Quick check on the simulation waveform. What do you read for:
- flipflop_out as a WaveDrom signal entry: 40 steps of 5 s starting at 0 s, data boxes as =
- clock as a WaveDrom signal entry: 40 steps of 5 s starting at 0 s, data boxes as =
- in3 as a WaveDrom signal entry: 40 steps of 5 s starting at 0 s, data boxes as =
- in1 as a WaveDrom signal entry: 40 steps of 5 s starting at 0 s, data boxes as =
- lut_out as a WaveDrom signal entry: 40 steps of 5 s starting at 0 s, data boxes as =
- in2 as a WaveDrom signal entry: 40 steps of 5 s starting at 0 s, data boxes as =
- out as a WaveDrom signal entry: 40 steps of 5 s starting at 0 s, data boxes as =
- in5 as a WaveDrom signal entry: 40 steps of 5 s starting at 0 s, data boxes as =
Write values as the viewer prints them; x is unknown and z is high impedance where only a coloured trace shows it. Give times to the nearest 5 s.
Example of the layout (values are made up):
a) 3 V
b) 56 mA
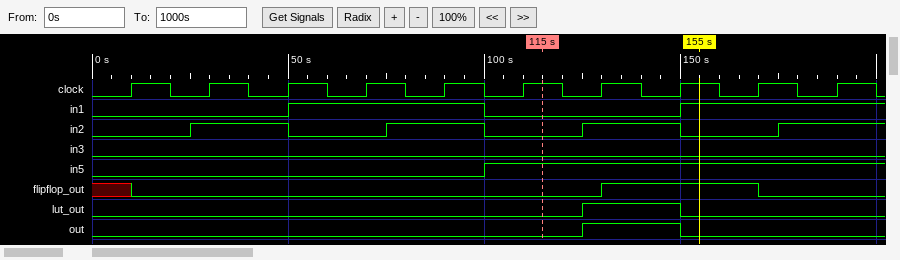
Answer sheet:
a) {name: 'flipflop_out', wave: 'x.0.......................1.......0.....'}
b) {name: 'clock', wave: '0.1.0.1.0.1.0.1.0.1.0.1.0.1.0.1.0.1.0.1.'}
c) {name: 'in3', wave: '0.......................................'}
d) {name: 'in1', wave: '0.........1.........0.........1.........'}
e) {name: 'lut_out', wave: '0........................1....0.........'}
f) {name: 'in2', wave: '0....1....0....1....0....1....0....1....'}
g) {name: 'out', wave: '0........................1....0.........'}
h) {name: 'in5', wave: '0...................1...................'}
